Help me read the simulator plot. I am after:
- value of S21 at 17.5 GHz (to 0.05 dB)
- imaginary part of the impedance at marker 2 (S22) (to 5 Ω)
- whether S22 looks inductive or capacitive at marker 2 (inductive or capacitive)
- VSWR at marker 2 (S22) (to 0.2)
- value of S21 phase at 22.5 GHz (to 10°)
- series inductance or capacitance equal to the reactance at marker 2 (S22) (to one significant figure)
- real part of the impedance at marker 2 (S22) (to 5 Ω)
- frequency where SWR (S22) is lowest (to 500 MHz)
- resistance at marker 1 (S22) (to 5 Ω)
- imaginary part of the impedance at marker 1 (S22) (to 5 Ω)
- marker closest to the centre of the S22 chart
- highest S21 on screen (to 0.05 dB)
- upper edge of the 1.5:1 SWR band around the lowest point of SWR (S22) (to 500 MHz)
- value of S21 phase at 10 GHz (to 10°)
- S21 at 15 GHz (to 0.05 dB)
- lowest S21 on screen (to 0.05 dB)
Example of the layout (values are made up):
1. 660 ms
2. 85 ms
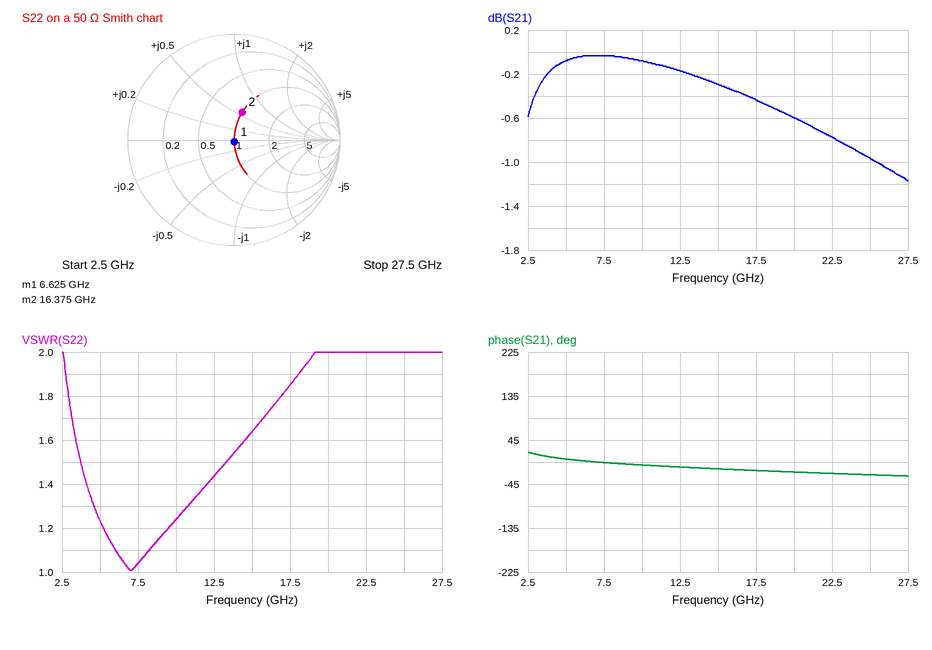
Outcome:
1. -0.45 dB
2. +30 Ω
3. inductive
4. 1.8
5. -20°
6. 300 pH
7. 50 Ω
8. 7.0 GHz
9. 50 Ω
10. 0 Ω
11. marker 1
12. -0.05 dB
13. 13.5 GHz
14. -10°
15. -0.30 dB
16. -1.15 dB
